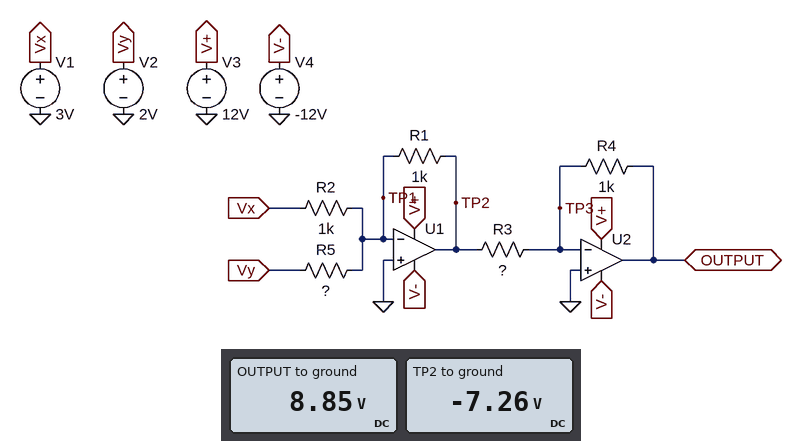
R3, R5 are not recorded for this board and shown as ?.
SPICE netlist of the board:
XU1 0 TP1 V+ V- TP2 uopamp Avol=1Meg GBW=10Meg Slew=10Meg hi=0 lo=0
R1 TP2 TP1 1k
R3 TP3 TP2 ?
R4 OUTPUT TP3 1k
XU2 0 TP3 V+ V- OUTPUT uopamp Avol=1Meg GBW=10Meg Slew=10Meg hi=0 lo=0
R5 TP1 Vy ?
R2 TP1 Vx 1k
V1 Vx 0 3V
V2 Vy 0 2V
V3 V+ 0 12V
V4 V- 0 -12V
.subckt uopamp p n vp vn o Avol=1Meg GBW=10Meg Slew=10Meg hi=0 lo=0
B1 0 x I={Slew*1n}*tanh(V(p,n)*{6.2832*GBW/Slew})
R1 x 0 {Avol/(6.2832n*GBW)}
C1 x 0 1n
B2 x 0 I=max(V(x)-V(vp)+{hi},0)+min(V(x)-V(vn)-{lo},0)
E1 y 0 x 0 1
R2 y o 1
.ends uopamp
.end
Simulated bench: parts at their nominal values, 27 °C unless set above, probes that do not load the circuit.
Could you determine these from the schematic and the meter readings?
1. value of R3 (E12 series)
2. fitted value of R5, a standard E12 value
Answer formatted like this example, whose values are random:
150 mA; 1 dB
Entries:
820 Ω; 470 Ω
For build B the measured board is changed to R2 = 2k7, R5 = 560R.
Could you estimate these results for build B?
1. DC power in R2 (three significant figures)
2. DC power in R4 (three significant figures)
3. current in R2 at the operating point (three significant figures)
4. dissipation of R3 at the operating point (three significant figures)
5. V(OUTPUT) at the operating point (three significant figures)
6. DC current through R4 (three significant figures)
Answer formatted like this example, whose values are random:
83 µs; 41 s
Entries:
3.33 mW; 32.6 mW; 1.11 mA; 26.7 mW; 5.71 V; 5.71 mA
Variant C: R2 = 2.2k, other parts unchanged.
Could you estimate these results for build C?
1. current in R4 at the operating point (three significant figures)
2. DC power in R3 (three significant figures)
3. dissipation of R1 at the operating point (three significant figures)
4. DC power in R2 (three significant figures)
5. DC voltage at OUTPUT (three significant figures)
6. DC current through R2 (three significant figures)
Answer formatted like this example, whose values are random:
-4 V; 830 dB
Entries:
6.85 mA; 38.5 mW; 31.6 mW; 4.09 mW; 6.85 V; 1.36 mA
